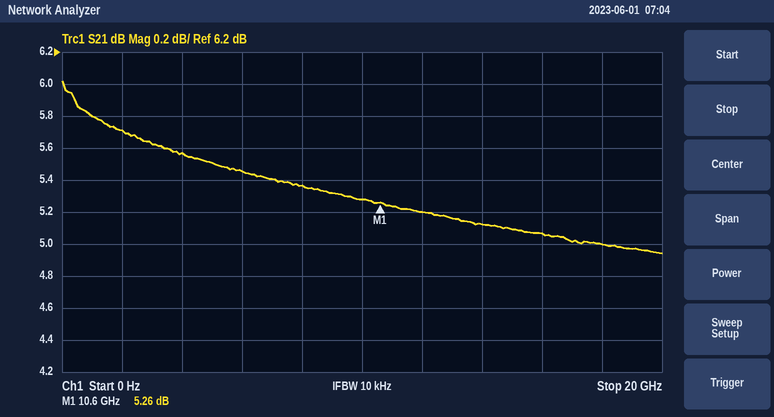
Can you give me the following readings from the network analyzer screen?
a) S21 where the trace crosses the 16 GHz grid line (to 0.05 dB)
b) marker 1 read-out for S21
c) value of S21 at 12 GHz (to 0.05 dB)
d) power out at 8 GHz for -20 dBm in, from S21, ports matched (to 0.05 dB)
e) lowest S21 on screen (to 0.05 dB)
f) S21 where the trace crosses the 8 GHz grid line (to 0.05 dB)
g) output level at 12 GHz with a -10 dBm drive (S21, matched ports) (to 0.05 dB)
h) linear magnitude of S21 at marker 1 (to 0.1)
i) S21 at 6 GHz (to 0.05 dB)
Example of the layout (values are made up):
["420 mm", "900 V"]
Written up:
["5.05 dB", "5.26 dB", "5.20 dB", "-14.65 dBm", "4.95 dB", "5.35 dB", "-4.80 dBm", "1.8", "5.45 dB"]
